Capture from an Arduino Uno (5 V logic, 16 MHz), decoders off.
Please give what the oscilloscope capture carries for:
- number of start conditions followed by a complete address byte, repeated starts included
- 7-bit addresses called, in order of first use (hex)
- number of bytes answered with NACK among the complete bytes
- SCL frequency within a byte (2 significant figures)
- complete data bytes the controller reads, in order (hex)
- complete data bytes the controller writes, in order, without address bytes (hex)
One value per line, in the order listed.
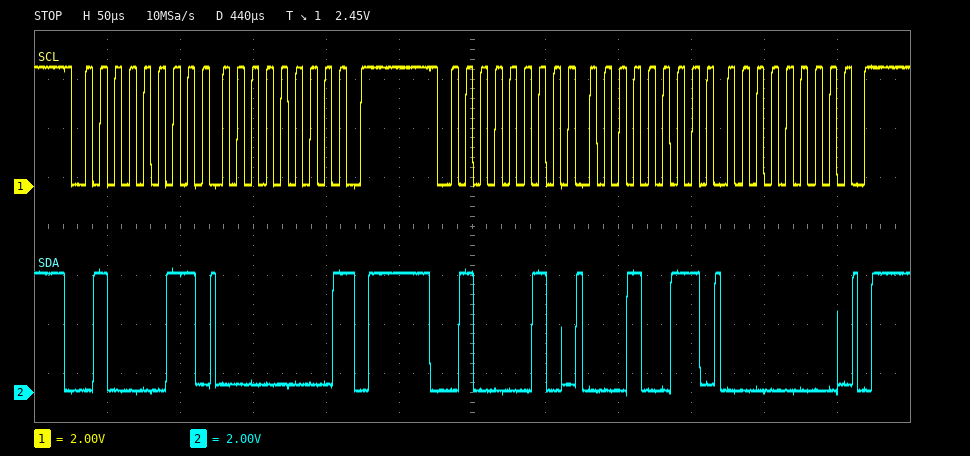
2
0x21
1
100 kHz
00
13 00
